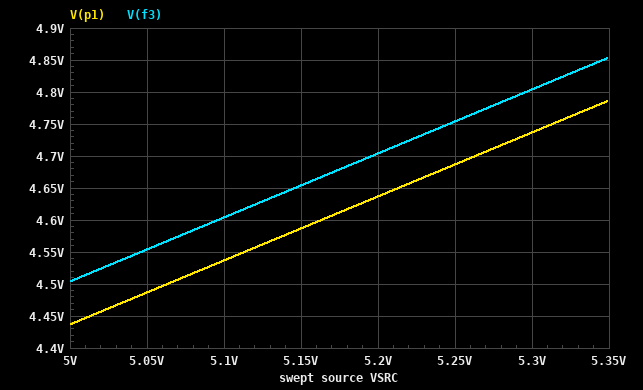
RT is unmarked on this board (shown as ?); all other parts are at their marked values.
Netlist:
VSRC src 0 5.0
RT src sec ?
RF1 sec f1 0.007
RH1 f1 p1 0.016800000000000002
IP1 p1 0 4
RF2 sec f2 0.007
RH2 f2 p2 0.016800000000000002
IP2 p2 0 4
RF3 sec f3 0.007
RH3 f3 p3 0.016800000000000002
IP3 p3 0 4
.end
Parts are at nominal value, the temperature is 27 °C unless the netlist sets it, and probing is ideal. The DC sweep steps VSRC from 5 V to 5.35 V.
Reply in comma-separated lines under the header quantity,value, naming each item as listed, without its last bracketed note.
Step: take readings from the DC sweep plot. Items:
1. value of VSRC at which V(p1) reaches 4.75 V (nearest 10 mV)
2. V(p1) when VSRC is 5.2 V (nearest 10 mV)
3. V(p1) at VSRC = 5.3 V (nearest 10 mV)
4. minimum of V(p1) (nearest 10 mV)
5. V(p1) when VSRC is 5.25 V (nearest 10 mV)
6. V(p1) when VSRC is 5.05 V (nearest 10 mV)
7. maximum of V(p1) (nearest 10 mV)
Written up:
quantity,value
value of VSRC at which V(p1) reaches 4.75 V,5.31 V
V(p1) when VSRC is 5.2 V,4.64 V
V(p1) at VSRC = 5.3 V,4.74 V
minimum of V(p1),4.44 V
V(p1) when VSRC is 5.25 V,4.69 V
V(p1) when VSRC is 5.05 V,4.49 V
maximum of V(p1),4.79 V
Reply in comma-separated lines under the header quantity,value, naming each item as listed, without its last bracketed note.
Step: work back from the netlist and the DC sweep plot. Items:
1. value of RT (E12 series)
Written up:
quantity,value
value of RT,0.039 Ω
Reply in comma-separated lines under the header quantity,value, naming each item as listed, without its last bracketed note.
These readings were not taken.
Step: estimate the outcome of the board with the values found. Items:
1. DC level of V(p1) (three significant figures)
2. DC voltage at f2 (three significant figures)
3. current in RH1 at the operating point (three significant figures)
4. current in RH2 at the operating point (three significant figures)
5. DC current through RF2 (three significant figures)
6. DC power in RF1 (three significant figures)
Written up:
quantity,value
DC level of V(p1),4.44 V
DC voltage at f2,4.50 V
current in RH1 at the operating point,4.00 A
current in RH2 at the operating point,4.00 A
DC current through RF2,4.00 A
DC power in RF1,112 mW
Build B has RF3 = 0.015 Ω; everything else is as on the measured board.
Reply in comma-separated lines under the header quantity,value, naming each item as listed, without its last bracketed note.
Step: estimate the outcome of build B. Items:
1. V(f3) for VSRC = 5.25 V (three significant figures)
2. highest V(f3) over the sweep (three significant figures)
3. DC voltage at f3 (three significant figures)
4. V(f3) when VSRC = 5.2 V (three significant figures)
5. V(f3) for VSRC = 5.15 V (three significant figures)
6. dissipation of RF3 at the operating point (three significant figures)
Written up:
quantity,value
V(f3) for VSRC = 5.25 V,4.72 V
highest V(f3) over the sweep,4.82 V
DC voltage at f3,4.47 V
V(f3) when VSRC = 5.2 V,4.67 V
V(f3) for VSRC = 5.15 V,4.62 V
dissipation of RF3 at the operating point,240 mW
